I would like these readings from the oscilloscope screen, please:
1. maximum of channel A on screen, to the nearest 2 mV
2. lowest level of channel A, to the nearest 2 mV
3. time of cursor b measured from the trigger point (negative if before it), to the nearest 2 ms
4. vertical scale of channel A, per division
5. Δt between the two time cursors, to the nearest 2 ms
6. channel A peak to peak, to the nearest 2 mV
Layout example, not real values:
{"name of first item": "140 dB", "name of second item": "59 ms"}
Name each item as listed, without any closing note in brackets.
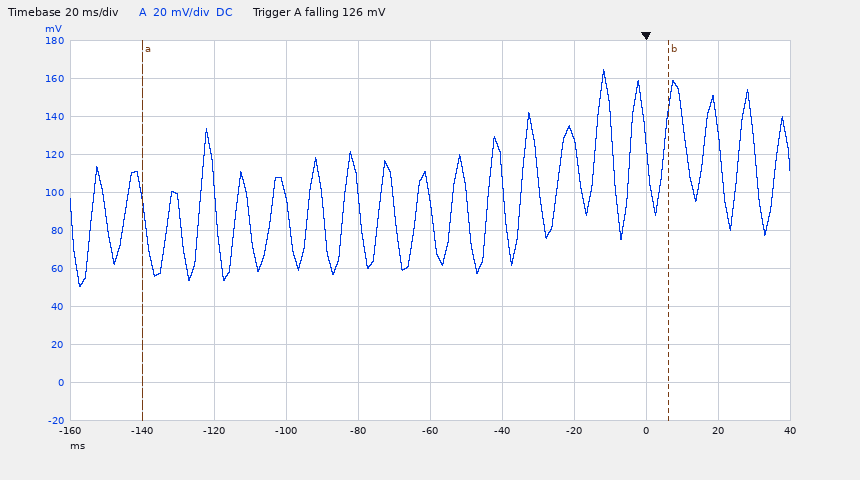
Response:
{"maximum of channel A on screen, to the nearest 2 mV": "164 mV", "lowest level of channel A, to the nearest 2 mV": "50 mV", "time of cursor b measured from the trigger point (negative if before it), to the nearest 2 ms": "+6 ms", "vertical scale of channel A, per division": "20 mV", "Δt between the two time cursors, to the nearest 2 ms": "146 ms", "channel A peak to peak, to the nearest 2 mV": "114 mV"}
